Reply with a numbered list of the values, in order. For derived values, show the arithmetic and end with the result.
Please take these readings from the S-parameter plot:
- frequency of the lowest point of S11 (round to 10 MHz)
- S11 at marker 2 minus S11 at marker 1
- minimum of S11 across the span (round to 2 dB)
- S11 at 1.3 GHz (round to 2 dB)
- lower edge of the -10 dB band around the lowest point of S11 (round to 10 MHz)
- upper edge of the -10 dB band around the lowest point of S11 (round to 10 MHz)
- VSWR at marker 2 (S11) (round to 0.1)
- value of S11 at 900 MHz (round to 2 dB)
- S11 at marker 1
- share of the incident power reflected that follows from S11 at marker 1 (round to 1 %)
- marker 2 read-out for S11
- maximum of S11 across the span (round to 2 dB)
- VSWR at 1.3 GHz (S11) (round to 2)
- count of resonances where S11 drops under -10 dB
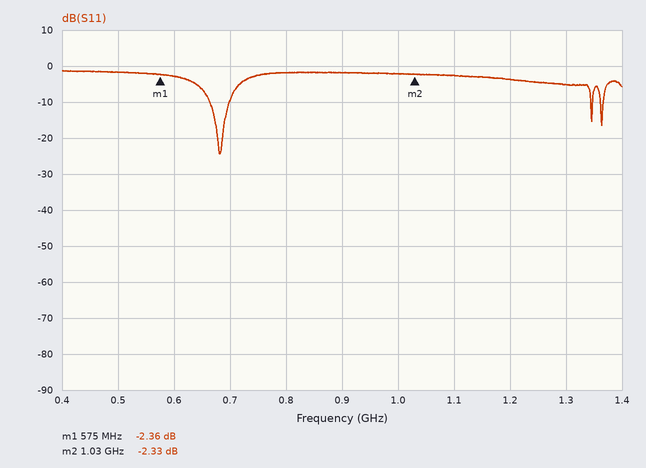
1. 680 MHz
2. -2.33 − (-2.36) = 0.03 dB
3. -24 dB
4. -6 dB
5. 660 MHz
6. 700 MHz
7. (1 + 0.7647)/(1 − 0.7647) ≈ 7.5
8. -2 dB
9. -2.36 dB
10. 10^(-2.36/10) ≈ 58 %
11. -2.33 dB
12. -2 dB
13. |Γ| = 10^(-6/20) = 0.5012; VSWR = (1 + 0.5012)/(1 − 0.5012) ≈ 3.01, so 4 to the nearest 2
14. 3
